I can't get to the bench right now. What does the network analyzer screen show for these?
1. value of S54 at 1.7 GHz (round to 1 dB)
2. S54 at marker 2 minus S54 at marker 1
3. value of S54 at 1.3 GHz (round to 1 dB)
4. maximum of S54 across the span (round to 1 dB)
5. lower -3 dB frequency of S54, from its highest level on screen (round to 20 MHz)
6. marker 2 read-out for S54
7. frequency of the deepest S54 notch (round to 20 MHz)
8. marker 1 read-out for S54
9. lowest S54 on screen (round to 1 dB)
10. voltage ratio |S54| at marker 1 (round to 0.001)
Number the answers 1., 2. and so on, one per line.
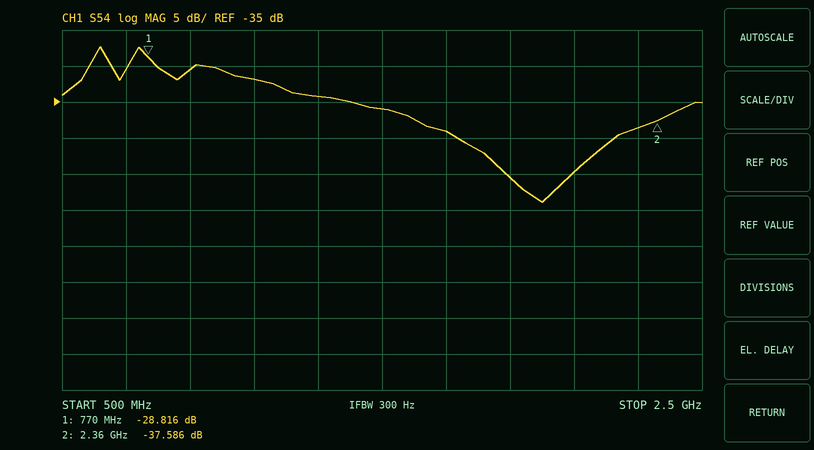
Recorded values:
1. -39 dB
2. -8.770 dB
3. -34 dB
4. -27 dB
5. 580 MHz
6. -37.586 dB
7. 2.00 GHz
8. -28.816 dB
9. -49 dB
10. 0.036
